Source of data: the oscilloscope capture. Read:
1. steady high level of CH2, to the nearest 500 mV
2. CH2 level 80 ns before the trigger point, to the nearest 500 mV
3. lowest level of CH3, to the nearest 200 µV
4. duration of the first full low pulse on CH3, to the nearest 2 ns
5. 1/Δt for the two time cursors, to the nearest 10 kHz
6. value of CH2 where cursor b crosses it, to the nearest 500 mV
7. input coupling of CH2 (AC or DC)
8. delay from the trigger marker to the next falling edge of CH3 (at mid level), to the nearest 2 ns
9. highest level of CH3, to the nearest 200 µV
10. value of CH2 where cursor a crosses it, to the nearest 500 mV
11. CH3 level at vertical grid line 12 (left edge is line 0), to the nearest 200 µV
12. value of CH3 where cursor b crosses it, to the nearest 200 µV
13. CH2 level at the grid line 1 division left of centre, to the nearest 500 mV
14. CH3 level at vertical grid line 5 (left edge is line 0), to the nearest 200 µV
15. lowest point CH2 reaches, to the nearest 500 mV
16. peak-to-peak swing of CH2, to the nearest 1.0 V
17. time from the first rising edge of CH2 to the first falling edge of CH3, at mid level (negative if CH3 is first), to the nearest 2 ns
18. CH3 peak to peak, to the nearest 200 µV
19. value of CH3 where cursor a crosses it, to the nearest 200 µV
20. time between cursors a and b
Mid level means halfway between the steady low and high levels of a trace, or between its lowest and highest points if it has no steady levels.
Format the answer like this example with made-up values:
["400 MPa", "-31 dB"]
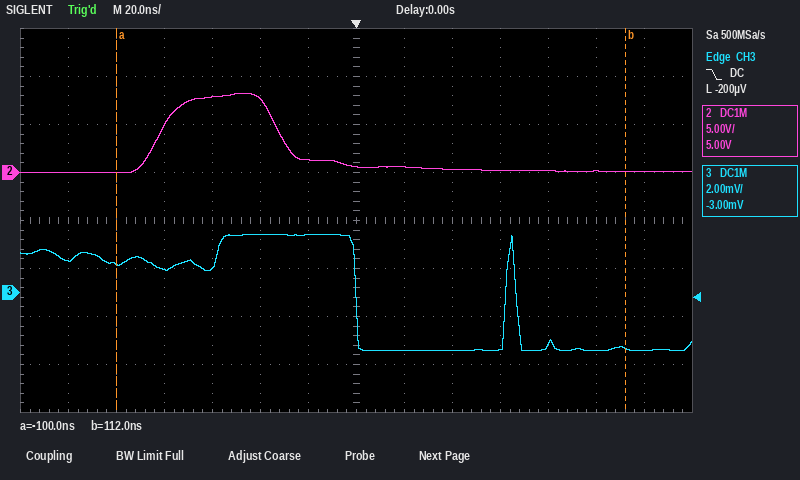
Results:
["8.0 V", "5.0 V", "-2.4 mV", "62 ns", "4.72 MHz", "0.0 V", "DC", "66 ns", "2.4 mV", "0.0 V", "-2.4 mV", "-2.4 mV", "1.5 V", "2.4 mV", "0.0 V", "8.0 V", "+82 ns", "4.8 mV", "1.2 mV", "212 ns"]
